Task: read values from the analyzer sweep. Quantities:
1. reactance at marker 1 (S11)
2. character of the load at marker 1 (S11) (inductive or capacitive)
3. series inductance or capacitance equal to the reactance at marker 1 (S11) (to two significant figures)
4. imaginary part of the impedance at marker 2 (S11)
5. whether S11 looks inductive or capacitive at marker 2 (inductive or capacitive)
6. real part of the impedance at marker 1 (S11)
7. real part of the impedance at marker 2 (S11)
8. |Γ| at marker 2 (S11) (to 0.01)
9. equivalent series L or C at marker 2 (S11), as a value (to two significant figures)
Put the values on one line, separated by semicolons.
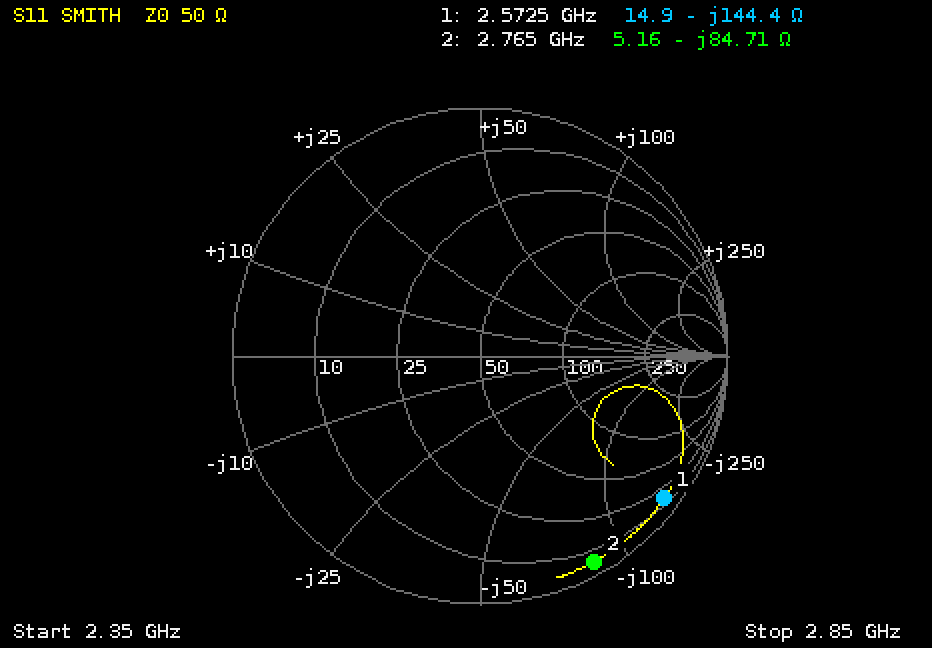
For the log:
-144.4 Ω; capacitive; 430 fF; -84.71 Ω; capacitive; 14.9 Ω; 5.16 Ω; 0.95; 680 fF
